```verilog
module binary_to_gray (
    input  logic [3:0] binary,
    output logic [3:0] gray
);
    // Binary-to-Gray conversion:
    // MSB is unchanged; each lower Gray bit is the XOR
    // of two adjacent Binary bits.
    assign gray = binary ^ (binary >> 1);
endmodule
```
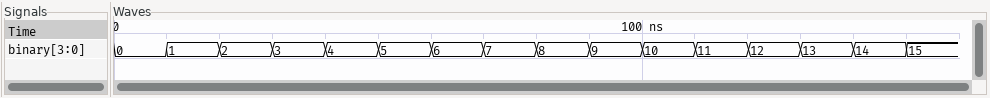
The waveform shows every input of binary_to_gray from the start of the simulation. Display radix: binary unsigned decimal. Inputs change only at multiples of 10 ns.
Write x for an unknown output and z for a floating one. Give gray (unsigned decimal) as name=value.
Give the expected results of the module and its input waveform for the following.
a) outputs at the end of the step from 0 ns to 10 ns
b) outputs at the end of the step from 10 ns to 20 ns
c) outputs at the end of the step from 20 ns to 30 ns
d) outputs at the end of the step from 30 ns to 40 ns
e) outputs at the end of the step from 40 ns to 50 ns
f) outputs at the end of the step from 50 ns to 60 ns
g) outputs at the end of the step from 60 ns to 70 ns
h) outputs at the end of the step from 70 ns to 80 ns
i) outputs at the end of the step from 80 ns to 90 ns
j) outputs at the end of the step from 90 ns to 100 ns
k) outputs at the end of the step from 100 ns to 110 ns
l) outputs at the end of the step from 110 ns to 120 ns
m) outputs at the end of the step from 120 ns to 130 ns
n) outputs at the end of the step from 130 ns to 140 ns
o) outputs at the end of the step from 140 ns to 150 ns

gray=0
gray=1
gray=3
gray=2
gray=6
gray=7
gray=5
gray=4
gray=12
gray=13
gray=15
gray=14
gray=10
gray=11
gray=9
